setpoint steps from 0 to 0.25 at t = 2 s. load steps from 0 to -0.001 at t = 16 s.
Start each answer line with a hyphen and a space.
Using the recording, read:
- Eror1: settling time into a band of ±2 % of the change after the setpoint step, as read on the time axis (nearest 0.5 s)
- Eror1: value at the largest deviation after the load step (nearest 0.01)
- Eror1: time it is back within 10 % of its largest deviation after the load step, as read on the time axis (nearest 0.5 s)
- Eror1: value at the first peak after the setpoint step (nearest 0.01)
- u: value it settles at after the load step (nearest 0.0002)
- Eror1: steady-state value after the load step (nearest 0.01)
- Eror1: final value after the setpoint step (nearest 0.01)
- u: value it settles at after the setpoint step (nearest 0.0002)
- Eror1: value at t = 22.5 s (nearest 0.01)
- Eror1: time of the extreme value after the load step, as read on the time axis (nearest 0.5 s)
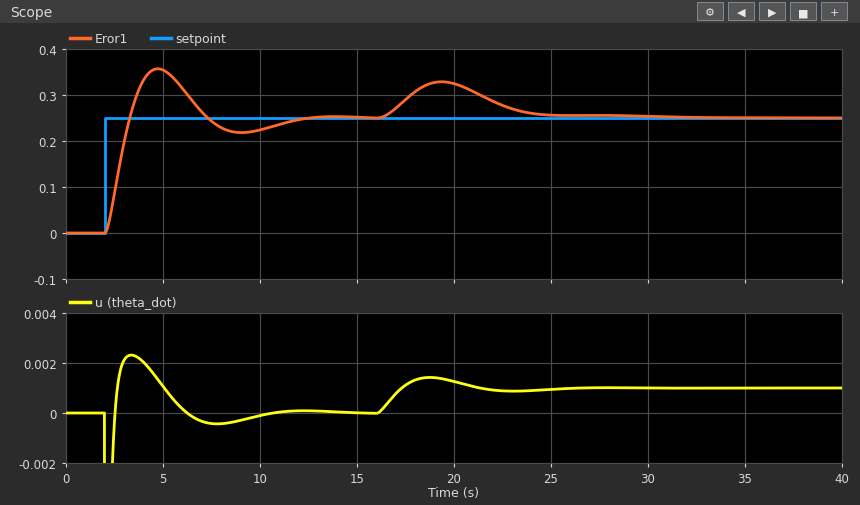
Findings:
- 12.0 s
- 0.33
- 24.5 s
- 0.36
- 0.0010
- 0.25
- 0.25
- 0.0000
- 0.28
- 19.5 s
